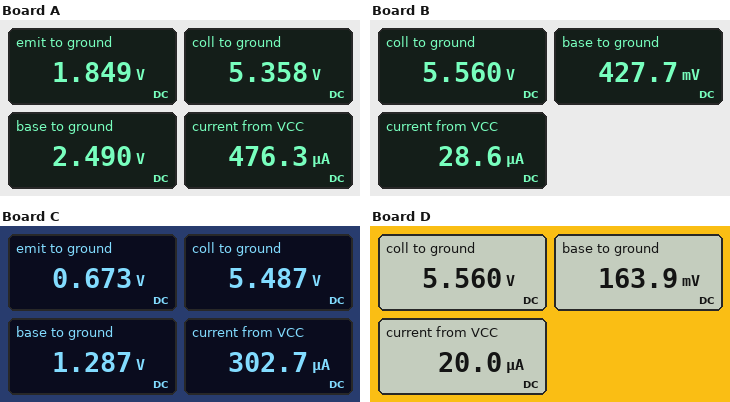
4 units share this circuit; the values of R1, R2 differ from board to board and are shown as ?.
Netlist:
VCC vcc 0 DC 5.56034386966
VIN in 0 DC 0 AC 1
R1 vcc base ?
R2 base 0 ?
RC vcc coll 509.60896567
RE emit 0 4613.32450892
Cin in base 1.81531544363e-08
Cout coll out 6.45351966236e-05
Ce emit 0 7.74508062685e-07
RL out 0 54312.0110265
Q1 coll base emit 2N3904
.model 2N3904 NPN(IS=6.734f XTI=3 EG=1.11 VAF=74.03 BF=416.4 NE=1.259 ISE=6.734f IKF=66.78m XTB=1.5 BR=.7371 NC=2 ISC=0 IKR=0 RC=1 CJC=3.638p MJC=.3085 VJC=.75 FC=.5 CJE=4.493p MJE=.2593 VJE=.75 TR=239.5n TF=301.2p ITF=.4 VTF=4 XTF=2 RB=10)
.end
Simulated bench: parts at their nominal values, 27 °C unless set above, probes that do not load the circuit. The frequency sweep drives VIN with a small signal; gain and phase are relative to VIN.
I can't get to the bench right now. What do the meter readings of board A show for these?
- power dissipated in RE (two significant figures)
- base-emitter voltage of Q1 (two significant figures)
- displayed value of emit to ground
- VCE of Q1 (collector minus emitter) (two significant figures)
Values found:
740 µW
640 mV
1.849 V
3.5 V
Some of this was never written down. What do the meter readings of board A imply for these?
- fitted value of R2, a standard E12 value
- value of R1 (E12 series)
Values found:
33 kΩ
39 kΩ
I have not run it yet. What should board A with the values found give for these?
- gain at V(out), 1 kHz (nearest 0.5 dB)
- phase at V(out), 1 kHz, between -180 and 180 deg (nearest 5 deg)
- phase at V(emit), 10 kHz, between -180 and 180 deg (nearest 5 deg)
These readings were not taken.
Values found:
4.5 dB
-85 deg
-65 deg
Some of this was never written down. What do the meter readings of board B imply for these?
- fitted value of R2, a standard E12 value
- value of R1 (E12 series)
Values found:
15 kΩ
180 kΩ
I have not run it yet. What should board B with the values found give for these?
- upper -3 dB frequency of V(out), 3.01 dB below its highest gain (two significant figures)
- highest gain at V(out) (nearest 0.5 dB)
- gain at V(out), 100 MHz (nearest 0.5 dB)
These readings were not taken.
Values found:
3.2 GHz
-0.5 dB
-5.5 dB
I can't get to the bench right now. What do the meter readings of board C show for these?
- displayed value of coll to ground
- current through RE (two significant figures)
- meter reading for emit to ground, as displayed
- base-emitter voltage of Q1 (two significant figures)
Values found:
5.487 V
150 µA
0.673 V
610 mV
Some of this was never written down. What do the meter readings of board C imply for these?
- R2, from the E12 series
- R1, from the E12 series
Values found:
8.2 kΩ
27 kΩ
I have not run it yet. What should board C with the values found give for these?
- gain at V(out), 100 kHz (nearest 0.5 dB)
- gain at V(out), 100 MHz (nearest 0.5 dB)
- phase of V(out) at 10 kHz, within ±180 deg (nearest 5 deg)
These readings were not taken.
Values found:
9.0 dB
7.5 dB
-165 deg
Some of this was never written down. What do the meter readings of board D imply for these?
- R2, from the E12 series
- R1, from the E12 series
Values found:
8.2 kΩ
270 kΩ
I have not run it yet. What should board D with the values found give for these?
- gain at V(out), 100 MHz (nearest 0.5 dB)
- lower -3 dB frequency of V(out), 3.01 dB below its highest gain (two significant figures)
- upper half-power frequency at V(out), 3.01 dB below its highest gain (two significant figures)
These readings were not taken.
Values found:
-6.0 dB
150 MHz
3.7 GHz
